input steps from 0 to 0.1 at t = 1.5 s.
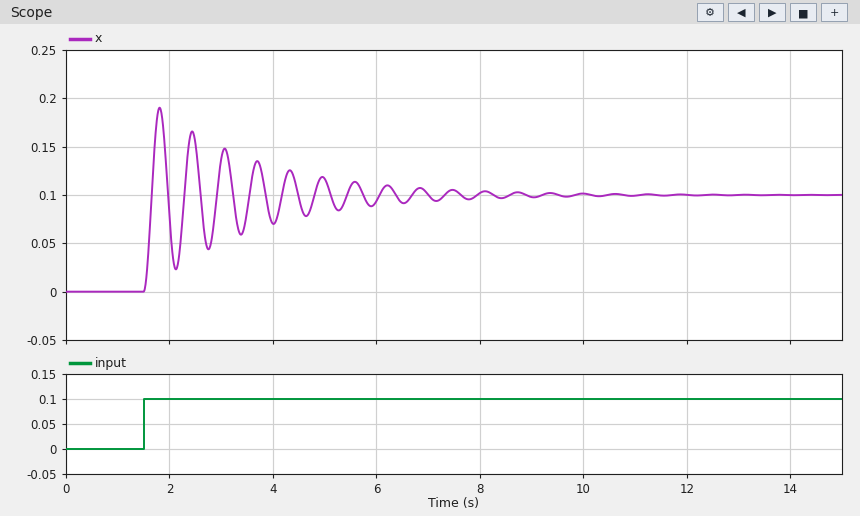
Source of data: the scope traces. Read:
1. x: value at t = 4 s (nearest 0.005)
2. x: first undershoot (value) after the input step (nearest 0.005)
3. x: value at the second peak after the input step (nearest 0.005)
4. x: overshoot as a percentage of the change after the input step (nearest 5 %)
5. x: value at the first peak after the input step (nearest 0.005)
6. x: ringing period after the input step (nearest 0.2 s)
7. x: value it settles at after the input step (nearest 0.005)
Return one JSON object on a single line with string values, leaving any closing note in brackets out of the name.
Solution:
{"x: value at t = 4 s": "0.070", "x: first undershoot (value) after the input step": "0.025", "x: value at the second peak after the input step": "0.165", "x: overshoot as a percentage of the change after the input step": "90 %", "x: value at the first peak after the input step": "0.190", "x: ringing period after the input step": "0.6 s", "x: value it settles at after the input step": "0.100"}
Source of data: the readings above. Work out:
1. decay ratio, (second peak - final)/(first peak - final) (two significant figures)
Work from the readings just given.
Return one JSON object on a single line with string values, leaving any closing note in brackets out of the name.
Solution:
{"decay ratio, (second peak - final)/(first peak - final)": "0.72"}
